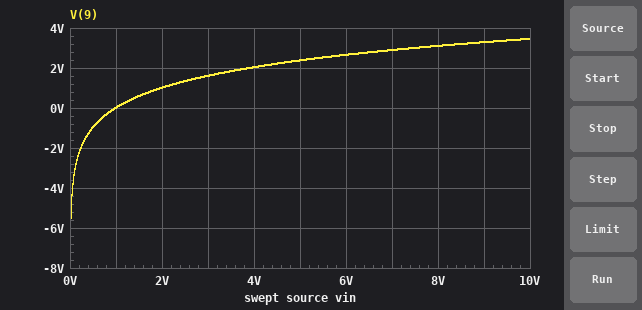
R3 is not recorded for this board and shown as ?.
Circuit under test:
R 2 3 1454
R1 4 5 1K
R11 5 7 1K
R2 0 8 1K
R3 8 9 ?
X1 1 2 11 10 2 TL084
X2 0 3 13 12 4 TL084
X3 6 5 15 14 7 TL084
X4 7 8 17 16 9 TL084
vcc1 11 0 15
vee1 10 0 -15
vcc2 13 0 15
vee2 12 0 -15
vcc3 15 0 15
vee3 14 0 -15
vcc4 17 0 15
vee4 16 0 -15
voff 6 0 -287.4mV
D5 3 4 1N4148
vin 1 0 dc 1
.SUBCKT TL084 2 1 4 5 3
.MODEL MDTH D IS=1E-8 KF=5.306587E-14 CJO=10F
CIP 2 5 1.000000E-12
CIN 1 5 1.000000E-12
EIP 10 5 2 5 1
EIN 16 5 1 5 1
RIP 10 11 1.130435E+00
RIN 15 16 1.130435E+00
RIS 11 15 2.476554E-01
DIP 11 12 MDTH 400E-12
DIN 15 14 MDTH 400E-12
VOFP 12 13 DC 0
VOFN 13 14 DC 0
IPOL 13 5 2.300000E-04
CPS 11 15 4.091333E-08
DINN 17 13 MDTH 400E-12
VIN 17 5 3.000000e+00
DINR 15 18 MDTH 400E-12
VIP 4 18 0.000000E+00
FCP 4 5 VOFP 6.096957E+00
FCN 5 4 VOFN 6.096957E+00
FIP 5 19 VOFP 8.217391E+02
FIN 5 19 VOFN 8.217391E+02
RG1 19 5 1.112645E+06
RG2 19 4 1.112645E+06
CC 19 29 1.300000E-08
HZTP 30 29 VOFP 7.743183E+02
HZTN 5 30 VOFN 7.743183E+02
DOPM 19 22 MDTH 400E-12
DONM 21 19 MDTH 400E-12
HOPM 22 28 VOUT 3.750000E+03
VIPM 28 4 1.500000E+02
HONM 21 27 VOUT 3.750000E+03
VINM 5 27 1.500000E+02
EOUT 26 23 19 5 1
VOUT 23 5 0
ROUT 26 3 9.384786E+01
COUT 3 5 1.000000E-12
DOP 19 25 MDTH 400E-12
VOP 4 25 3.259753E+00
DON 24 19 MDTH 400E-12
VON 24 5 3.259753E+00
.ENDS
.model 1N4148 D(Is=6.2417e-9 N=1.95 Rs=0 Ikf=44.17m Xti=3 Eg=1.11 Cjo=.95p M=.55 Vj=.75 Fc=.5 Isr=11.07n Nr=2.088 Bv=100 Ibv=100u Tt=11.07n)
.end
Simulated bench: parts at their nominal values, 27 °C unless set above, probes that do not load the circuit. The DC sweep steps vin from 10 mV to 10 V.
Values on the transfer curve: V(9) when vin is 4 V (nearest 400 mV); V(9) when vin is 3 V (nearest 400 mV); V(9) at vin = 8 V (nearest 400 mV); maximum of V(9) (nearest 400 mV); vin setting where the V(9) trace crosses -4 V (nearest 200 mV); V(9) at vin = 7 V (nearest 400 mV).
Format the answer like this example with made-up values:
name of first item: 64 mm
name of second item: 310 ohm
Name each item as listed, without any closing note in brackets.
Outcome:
V(9) when vin is 4 V: 2.0 V
V(9) when vin is 3 V: 1.6 V
V(9) at vin = 8 V: 3.2 V
maximum of V(9): 3.6 V
vin setting where the V(9) trace crosses -4 V: 0 V
V(9) at vin = 7 V: 2.8 V
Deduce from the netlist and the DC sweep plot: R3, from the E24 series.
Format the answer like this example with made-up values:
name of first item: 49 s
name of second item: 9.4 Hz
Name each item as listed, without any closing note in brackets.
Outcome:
R3, from the E24 series: 24 kΩ
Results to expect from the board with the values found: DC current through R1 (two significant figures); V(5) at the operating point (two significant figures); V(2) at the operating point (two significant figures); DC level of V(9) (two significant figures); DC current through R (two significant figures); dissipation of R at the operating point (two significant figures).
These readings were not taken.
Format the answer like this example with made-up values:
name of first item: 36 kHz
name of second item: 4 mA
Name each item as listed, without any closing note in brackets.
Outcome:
DC current through R1: 290 µA
V(5) at the operating point: -290 mV
V(2) at the operating point: 1.0 V
DC level of V(9): 17 mV
DC current through R: 690 µA
dissipation of R at the operating point: 690 µW
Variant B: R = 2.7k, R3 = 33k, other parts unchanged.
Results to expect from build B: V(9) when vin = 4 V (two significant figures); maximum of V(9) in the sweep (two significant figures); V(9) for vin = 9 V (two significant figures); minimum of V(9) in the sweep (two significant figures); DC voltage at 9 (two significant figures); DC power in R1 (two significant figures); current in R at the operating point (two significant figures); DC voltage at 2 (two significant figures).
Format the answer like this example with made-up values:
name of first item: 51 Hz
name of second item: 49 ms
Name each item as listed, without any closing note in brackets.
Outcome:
V(9) when vin = 4 V: 1.5 V
maximum of V(9) in the sweep: 3.4 V
V(9) for vin = 9 V: 3.2 V
minimum of V(9) in the sweep: -9.7 V
DC voltage at 9: -1.2 V
DC power in R1: 64 µW
current in R at the operating point: 370 µA
DC voltage at 2: 1.0 V
